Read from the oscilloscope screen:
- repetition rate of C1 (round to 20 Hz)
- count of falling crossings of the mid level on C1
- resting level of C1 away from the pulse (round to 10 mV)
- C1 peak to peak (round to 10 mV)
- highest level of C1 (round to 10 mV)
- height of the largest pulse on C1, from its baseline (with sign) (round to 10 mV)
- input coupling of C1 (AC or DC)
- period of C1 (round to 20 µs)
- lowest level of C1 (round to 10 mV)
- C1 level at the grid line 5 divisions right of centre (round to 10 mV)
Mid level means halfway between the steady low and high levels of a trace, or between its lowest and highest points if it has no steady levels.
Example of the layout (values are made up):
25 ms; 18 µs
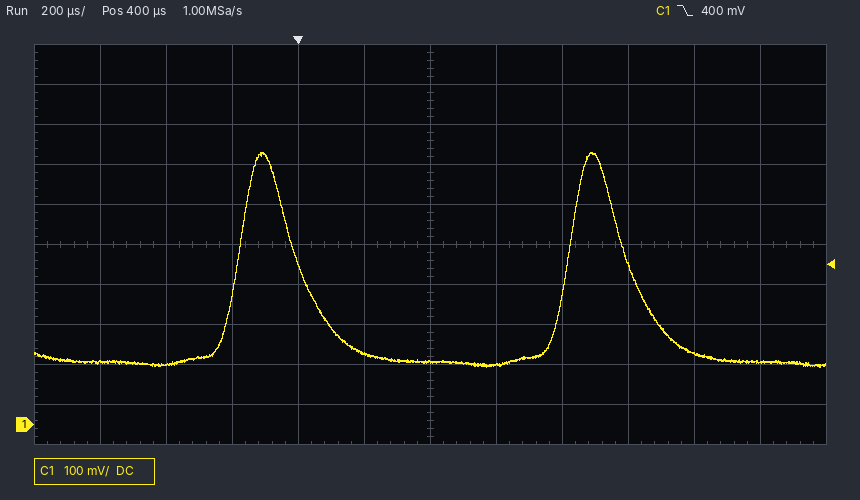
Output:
1.00 kHz; 2; 160 mV; 540 mV; 680 mV; +520 mV; DC; 1.00 ms; 140 mV; 160 mV
